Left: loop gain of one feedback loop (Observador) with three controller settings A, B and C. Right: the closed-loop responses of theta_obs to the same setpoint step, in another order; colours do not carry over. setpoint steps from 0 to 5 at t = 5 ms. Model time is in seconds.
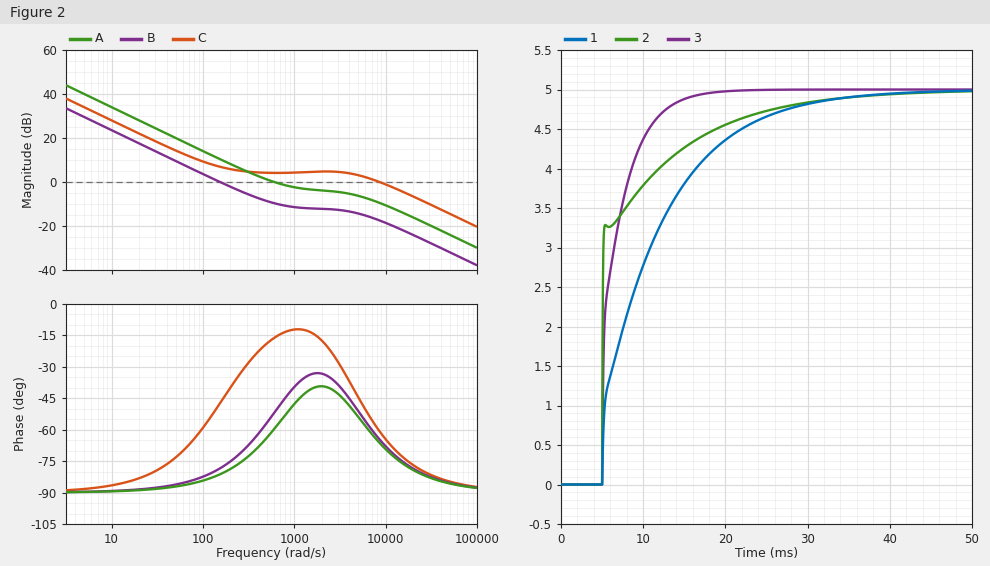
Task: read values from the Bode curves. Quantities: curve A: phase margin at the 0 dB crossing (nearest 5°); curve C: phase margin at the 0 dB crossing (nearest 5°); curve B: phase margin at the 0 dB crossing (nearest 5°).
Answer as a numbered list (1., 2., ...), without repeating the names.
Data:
1. 120°
2. 120°
3. 100°
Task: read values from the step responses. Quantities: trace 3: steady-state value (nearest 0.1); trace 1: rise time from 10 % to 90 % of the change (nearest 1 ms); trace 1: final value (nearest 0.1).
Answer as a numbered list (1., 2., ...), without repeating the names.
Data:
1. 5.0
2. 17 ms
3. 5.0
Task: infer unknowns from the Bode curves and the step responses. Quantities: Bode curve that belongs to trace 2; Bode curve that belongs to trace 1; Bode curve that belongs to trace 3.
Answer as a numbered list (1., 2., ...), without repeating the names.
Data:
1. C
2. B
3. A
